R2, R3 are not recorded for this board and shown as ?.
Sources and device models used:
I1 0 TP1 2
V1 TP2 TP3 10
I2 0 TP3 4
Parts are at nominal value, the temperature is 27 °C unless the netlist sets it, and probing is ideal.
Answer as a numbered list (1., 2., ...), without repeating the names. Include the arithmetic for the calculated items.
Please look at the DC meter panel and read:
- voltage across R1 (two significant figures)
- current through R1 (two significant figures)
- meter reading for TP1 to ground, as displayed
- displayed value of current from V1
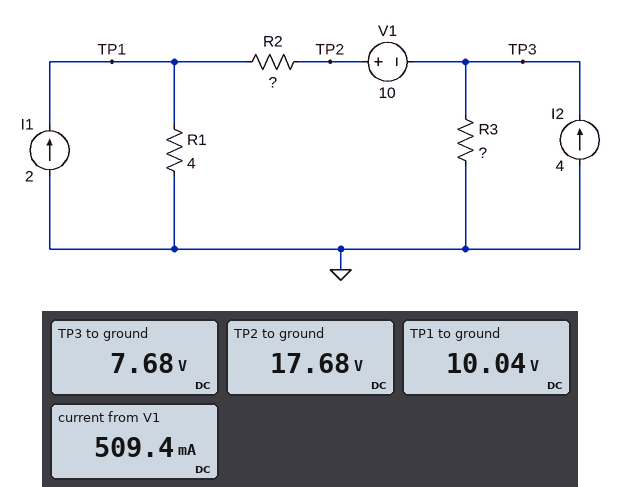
1. 10.04 V = 10 V
2. (10.04 V) / 4 Ω = 2.5 A
3. 10.04 V
4. 509.4 mA
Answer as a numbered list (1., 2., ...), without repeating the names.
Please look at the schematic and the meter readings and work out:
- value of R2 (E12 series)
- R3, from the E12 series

1. 15 Ω
2. 2.2 Ω
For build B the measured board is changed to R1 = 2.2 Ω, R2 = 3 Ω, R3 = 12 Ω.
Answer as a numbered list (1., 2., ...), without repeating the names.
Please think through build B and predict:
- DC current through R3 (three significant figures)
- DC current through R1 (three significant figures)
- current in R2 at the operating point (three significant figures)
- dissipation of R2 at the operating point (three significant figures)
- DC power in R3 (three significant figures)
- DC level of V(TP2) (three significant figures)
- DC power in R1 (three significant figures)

1. 884 mA
2. 5.12 A
3. 3.12 A
4. 29.1 W
5. 9.37 W
6. 20.6 V
7. 57.6 W
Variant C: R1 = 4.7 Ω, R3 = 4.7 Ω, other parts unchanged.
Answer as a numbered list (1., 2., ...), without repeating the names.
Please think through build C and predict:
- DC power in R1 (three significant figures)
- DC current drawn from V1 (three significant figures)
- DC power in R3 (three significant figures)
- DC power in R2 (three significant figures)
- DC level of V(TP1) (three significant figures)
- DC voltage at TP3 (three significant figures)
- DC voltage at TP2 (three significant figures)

1. 36.7 W
2. 795 mA
3. 48.3 W
4. 9.48 W
5. 13.1 V
6. 15.1 V
7. 25.1 V
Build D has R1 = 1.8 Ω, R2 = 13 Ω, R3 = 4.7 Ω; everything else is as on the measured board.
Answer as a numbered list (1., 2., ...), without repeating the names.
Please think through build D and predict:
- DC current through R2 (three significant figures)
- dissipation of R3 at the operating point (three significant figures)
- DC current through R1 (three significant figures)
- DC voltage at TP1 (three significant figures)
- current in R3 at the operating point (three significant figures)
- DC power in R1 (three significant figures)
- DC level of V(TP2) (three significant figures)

1. 1.29 A
2. 34.5 W
3. 3.29 A
4. 5.93 V
5. 2.71 A
6. 19.5 W
7. 22.7 V
